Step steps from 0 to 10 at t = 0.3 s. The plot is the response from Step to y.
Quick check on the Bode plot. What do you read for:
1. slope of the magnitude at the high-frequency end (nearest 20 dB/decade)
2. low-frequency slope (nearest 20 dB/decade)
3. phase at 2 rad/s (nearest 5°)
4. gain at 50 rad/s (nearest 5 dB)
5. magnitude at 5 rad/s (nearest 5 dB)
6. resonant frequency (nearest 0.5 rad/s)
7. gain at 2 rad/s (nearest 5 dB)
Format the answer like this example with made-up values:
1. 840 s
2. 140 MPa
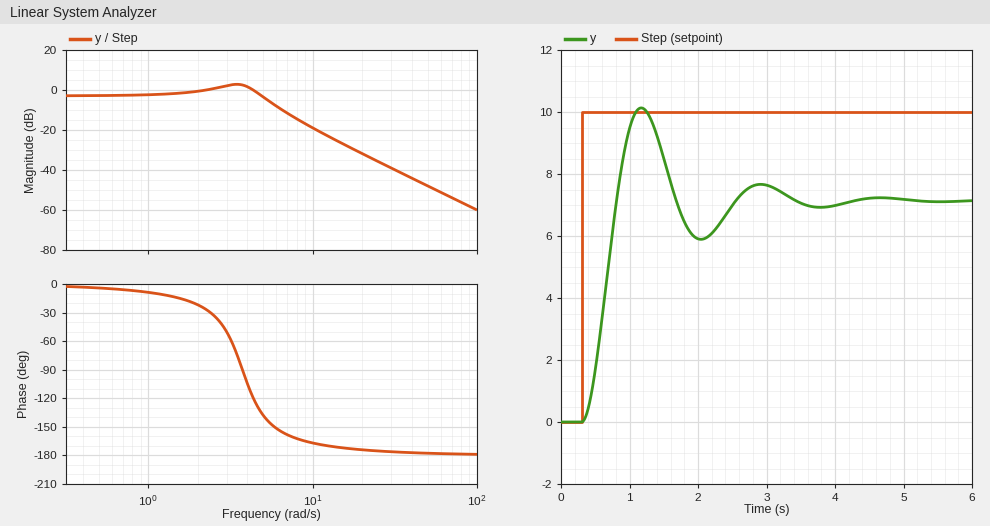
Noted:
1. -40 dB/decade
2. 0 dB/decade
3. -20°
4. -50 dB
5. -5 dB
6. 3.5 rad/s
7. 0 dB
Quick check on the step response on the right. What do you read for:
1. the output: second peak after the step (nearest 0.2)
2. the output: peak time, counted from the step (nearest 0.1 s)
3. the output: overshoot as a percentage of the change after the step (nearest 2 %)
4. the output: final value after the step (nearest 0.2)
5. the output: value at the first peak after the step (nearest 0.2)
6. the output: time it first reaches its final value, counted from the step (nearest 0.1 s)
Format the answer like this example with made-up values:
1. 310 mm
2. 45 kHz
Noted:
1. 7.6
2. 0.9 s
3. 42 %
4. 7.2
5. 10.2
6. 0.5 s
